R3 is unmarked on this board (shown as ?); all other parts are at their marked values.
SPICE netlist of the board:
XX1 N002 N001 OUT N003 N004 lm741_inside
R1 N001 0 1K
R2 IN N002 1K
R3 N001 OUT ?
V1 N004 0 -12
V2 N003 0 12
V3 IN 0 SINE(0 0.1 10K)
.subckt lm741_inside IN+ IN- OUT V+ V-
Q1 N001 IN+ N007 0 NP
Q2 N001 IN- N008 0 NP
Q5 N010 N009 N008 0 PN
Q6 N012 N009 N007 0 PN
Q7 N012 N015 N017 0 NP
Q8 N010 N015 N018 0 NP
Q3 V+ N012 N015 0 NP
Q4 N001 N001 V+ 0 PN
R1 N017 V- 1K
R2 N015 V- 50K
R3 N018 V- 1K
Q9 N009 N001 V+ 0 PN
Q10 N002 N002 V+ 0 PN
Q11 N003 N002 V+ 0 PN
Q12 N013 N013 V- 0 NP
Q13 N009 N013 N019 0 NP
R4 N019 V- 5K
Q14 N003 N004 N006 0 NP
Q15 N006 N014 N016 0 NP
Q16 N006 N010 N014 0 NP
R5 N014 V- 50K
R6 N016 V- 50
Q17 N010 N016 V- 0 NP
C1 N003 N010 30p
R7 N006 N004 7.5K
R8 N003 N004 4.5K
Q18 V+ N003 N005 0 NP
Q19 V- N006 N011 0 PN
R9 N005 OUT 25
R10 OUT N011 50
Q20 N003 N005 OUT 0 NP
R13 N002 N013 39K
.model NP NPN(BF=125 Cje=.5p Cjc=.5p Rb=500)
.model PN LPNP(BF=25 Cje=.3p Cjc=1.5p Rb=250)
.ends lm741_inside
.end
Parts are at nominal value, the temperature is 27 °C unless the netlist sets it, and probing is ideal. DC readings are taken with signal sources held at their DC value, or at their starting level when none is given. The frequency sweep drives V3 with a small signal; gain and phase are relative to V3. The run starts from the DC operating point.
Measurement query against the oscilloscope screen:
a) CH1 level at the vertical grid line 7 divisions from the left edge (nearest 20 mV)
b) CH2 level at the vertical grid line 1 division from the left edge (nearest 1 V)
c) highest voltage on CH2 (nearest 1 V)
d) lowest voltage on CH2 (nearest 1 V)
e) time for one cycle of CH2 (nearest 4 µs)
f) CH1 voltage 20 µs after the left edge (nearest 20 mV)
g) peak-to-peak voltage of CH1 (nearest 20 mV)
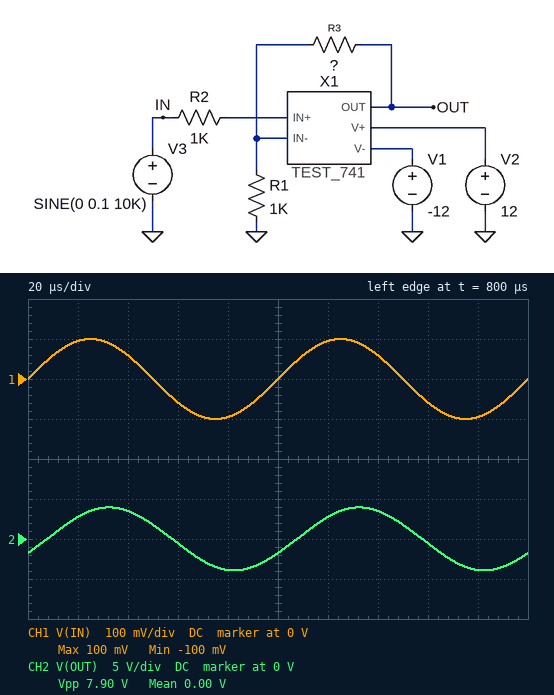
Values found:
60 mV
3 V
4 V
-4 V
100 µs
100 mV
200 mV
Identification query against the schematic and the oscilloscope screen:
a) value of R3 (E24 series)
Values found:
43 kΩ
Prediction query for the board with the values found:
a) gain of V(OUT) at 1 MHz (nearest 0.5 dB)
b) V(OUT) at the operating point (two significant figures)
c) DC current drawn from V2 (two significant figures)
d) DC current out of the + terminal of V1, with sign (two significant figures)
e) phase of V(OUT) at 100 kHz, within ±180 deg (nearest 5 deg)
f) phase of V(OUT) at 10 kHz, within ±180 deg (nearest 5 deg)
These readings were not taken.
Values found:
-2.0 dB
13 mV
1.2 mA
-1.2 mA
-80 deg
-30 deg
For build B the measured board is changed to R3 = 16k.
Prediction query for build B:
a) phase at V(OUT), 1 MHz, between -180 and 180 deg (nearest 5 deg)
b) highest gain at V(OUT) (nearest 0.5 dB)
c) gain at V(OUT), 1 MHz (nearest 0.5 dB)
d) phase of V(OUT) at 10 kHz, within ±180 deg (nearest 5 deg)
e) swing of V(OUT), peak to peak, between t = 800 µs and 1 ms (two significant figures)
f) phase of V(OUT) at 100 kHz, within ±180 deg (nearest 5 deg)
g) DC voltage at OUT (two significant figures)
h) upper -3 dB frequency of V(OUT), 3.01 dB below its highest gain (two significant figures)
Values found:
-90 deg
24.5 dB
-3.5 dB
-15 deg
3.3 V
-70 deg
4.9 mV
39 kHz
